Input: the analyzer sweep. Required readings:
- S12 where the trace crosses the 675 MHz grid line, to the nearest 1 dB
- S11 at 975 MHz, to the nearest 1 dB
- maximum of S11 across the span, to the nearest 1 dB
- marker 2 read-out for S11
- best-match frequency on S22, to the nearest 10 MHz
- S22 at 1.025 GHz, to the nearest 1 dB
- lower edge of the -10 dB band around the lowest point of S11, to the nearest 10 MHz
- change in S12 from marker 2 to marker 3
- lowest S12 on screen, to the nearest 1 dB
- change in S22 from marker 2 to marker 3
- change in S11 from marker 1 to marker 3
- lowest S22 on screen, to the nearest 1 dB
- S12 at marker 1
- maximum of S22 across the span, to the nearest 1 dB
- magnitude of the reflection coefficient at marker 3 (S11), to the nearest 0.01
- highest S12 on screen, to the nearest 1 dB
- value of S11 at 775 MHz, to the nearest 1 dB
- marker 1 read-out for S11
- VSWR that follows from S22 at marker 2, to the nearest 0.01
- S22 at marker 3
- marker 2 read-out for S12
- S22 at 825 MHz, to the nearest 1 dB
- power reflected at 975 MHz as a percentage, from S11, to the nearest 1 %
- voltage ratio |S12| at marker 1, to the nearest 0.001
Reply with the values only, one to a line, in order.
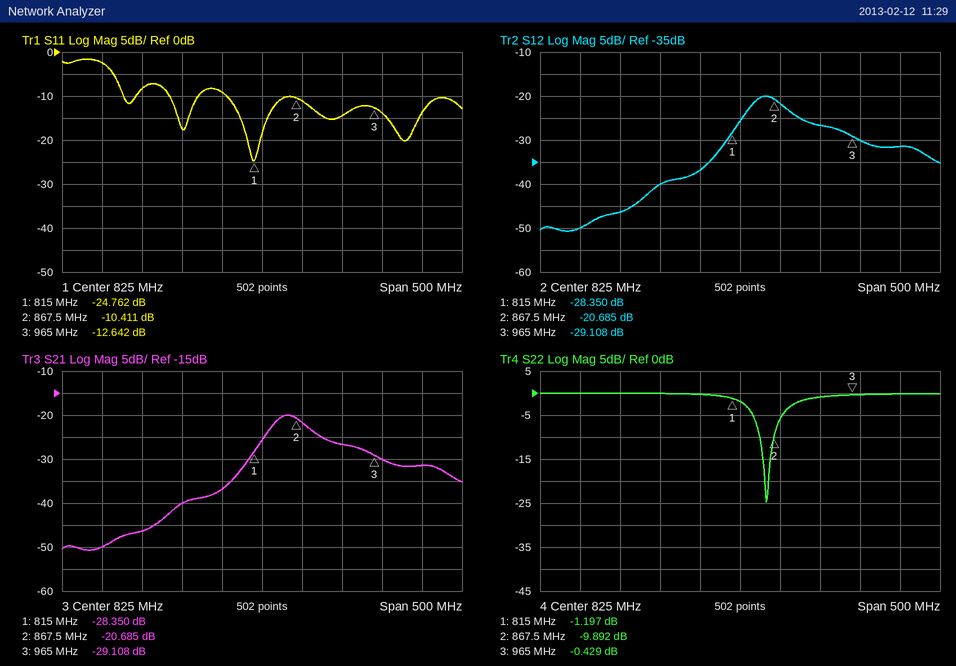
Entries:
-46 dB
-14 dB
-2 dB
-10.411 dB
860 MHz
0 dB
780 MHz
-8.423 dB
-51 dB
9.463 dB
12.120 dB
-25 dB
-28.350 dB
0 dB
0.23
-20 dB
-9 dB
-24.762 dB
1.94
-0.429 dB
-20.685 dB
-2 dB
4 %
0.038
